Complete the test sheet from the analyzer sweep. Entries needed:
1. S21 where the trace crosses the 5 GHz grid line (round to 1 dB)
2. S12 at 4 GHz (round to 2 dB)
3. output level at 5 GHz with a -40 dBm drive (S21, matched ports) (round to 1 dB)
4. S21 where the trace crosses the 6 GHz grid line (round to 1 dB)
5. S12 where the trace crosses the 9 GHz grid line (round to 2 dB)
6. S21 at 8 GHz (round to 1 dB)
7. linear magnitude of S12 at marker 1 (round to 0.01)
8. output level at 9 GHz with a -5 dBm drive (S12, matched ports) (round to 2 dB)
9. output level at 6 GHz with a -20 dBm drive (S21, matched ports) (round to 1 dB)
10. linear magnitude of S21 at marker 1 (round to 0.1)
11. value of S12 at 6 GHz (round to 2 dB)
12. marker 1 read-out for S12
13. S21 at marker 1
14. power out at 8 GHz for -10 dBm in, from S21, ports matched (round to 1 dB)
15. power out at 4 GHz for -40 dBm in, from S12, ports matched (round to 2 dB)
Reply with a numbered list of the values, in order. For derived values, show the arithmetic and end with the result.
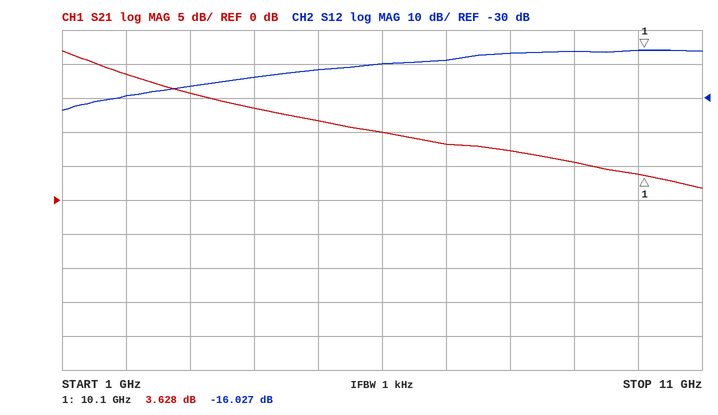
1. 12 dB
2. -24 dB
3. -40 dBm + (12 dB) = -28 dBm
4. 10 dB
5. -16 dB
6. 7 dB
7. 10^(-16.027/20) ≈ 0.16
8. -5 dBm + (-16 dB) = -22 dBm
9. -20 dBm + (10 dB) = -10 dBm
10. 10^(3.628/20) ≈ 1.5
11. -20 dB
12. -16.027 dB
13. 3.628 dB
14. -10 dBm + (7 dB) = -3 dBm
15. -40 dBm + (-24 dB) = -64 dBm
